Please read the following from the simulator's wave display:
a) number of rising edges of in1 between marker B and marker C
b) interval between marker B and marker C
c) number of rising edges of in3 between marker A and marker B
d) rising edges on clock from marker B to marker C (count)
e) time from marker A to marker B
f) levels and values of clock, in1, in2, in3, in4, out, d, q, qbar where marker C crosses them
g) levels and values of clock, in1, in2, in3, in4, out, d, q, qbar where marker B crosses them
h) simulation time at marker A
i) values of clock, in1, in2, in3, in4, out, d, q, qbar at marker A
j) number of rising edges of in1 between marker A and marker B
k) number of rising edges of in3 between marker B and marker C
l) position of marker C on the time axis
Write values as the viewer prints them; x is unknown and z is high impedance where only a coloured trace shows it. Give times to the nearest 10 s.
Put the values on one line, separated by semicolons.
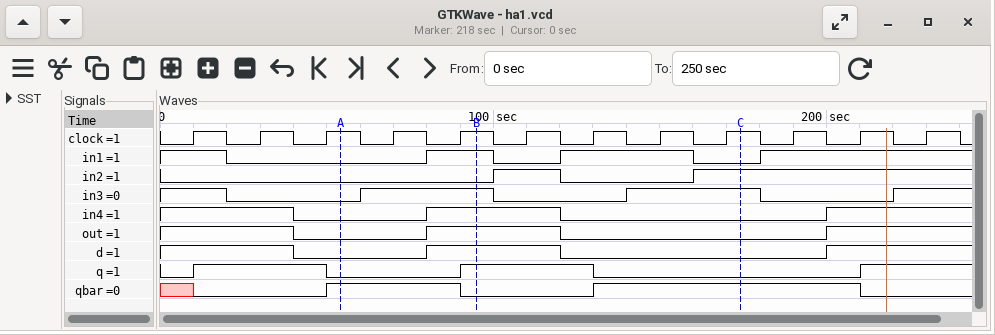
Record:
1; 80 s; 1; 4; 40 s; clock=1, in1=0, in2=1, in3=1, in4=0, out=0, d=0, q=0, qbar=1; clock=1, in1=1, in2=0, in3=1, in4=1, out=1, d=1, q=1, qbar=0; 50 s; clock=1, in1=0, in2=0, in3=0, in4=0, out=0, d=0, q=0, qbar=1; 1; 1; 170 s
